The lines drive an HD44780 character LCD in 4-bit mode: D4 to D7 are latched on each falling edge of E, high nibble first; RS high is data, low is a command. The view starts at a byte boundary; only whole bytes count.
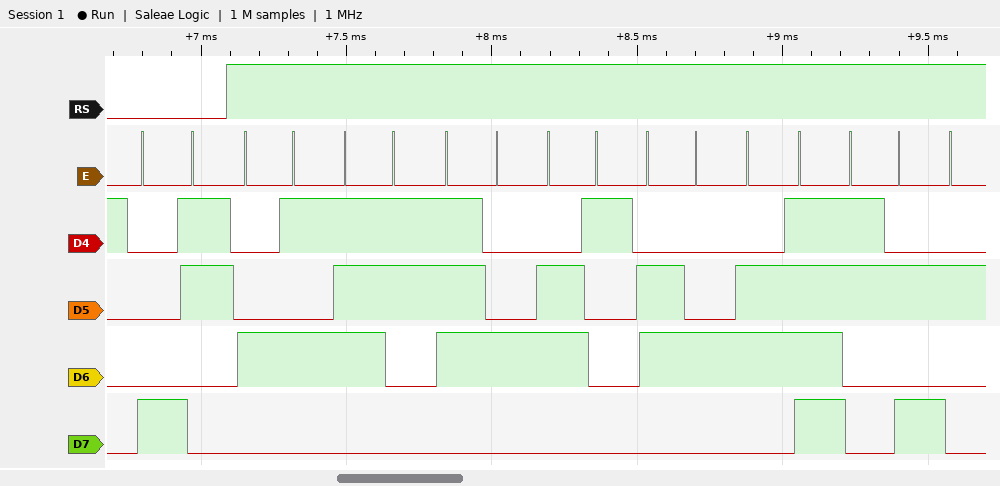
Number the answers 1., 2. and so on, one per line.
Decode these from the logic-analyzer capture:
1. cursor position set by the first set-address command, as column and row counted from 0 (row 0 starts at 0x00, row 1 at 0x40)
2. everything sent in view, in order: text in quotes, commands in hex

1. column 3, row 0
2. 0x83 "Estado:"
